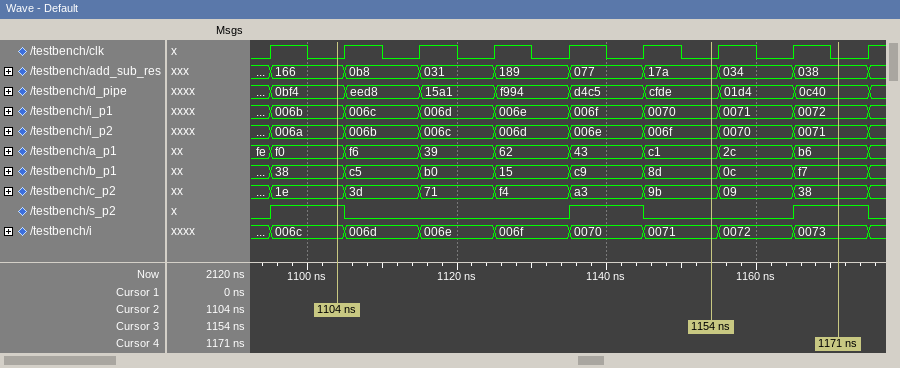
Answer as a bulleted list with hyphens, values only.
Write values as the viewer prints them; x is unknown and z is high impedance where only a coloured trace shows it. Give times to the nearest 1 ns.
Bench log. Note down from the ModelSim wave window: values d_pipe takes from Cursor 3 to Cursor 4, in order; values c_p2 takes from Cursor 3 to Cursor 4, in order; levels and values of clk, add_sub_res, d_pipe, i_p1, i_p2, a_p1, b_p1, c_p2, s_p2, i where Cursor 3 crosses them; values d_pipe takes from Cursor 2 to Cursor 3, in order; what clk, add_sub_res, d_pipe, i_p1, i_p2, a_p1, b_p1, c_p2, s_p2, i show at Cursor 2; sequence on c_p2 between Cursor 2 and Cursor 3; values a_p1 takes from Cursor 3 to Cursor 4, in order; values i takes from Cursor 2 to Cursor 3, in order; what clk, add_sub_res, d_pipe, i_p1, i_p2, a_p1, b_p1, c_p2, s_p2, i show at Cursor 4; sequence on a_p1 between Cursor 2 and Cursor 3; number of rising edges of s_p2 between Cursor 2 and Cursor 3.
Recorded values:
- cfde, 01d4, 0c40
- 9b, 09, 38
- clk=0, add_sub_res=17a, d_pipe=cfde, i_p1=0070, i_p2=006f, a_p1=c1, b_p1=8d, c_p2=9b, s_p2=0, i=0071
- 0bf4, eed8, 15a1, f994, d4c5, cfde
- clk=0, add_sub_res=166, d_pipe=0bf4, i_p1=006b, i_p2=006a, a_p1=f0, b_p1=38, c_p2=1e, s_p2=1, i=006c
- 1e, 3d, 71, f4, a3, 9b
- c1, 2c, b6
- 006c, 006d, 006e, 006f, 0070, 0071
- clk=0, add_sub_res=038, d_pipe=0c40, i_p1=0072, i_p2=0071, a_p1=b6, b_p1=f7, c_p2=38, s_p2=1, i=0073
- f0, f6, 39, 62, 43, c1
- 1
